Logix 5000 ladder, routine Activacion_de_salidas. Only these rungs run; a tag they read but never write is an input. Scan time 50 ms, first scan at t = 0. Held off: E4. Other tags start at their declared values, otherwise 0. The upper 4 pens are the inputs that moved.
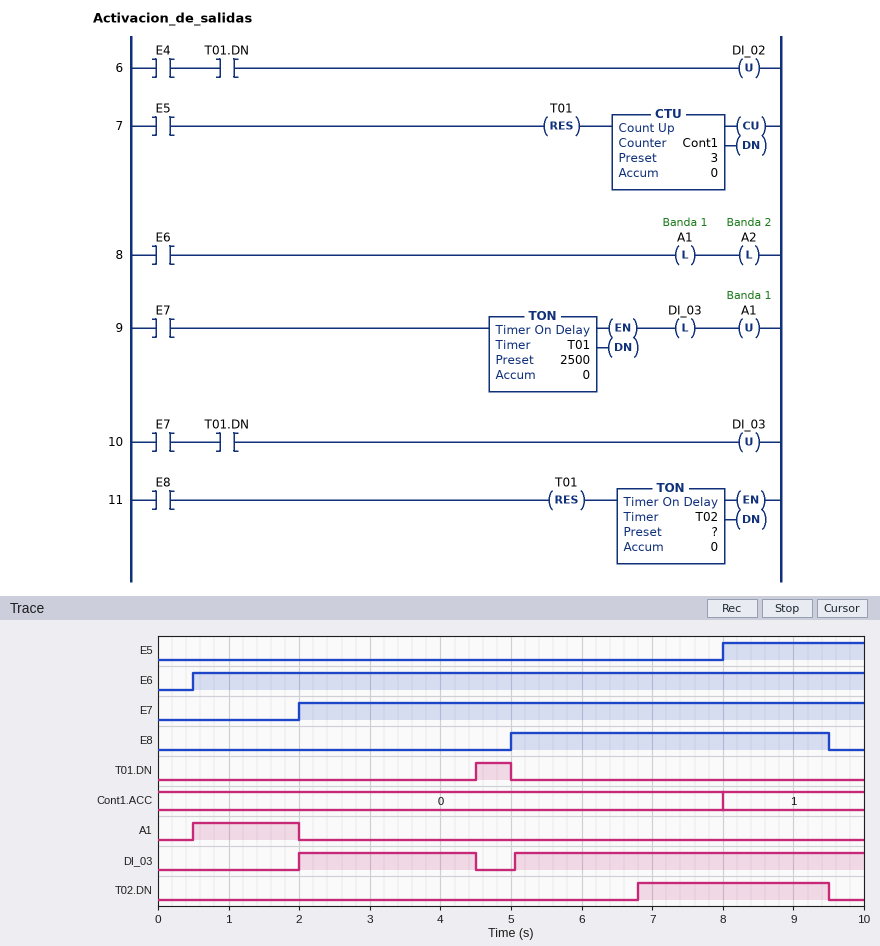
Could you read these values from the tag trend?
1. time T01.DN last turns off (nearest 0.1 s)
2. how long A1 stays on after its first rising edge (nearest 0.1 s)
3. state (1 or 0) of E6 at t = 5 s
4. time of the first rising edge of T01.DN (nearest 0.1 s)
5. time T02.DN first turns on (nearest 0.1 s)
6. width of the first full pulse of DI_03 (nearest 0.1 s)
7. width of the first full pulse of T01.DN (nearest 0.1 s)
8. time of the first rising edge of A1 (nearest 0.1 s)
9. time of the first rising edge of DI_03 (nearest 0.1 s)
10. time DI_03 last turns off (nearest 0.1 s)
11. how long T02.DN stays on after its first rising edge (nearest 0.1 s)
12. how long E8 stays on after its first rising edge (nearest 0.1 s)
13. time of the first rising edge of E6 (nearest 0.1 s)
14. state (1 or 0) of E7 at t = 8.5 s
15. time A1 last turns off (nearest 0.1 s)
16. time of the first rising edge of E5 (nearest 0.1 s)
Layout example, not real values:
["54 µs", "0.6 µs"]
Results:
["5.0 s", "1.5 s", "1", "4.5 s", "6.8 s", "2.5 s", "0.5 s", "0.5 s", "2.0 s", "4.5 s", "2.7 s", "4.5 s", "0.5 s", "1", "2.0 s", "8.0 s"]
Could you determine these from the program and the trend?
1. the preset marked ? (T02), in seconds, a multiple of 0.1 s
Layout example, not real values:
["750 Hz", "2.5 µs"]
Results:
["1.8 s"]
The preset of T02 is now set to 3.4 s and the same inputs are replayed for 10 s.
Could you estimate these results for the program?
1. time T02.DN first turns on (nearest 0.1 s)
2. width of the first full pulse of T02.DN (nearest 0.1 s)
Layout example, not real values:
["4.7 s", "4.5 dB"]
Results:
["8.4 s", "1.1 s"]
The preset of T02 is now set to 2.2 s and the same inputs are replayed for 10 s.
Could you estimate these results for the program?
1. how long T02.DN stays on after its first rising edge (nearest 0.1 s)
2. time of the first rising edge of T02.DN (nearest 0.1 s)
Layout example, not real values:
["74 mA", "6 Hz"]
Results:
["2.3 s", "7.2 s"]
